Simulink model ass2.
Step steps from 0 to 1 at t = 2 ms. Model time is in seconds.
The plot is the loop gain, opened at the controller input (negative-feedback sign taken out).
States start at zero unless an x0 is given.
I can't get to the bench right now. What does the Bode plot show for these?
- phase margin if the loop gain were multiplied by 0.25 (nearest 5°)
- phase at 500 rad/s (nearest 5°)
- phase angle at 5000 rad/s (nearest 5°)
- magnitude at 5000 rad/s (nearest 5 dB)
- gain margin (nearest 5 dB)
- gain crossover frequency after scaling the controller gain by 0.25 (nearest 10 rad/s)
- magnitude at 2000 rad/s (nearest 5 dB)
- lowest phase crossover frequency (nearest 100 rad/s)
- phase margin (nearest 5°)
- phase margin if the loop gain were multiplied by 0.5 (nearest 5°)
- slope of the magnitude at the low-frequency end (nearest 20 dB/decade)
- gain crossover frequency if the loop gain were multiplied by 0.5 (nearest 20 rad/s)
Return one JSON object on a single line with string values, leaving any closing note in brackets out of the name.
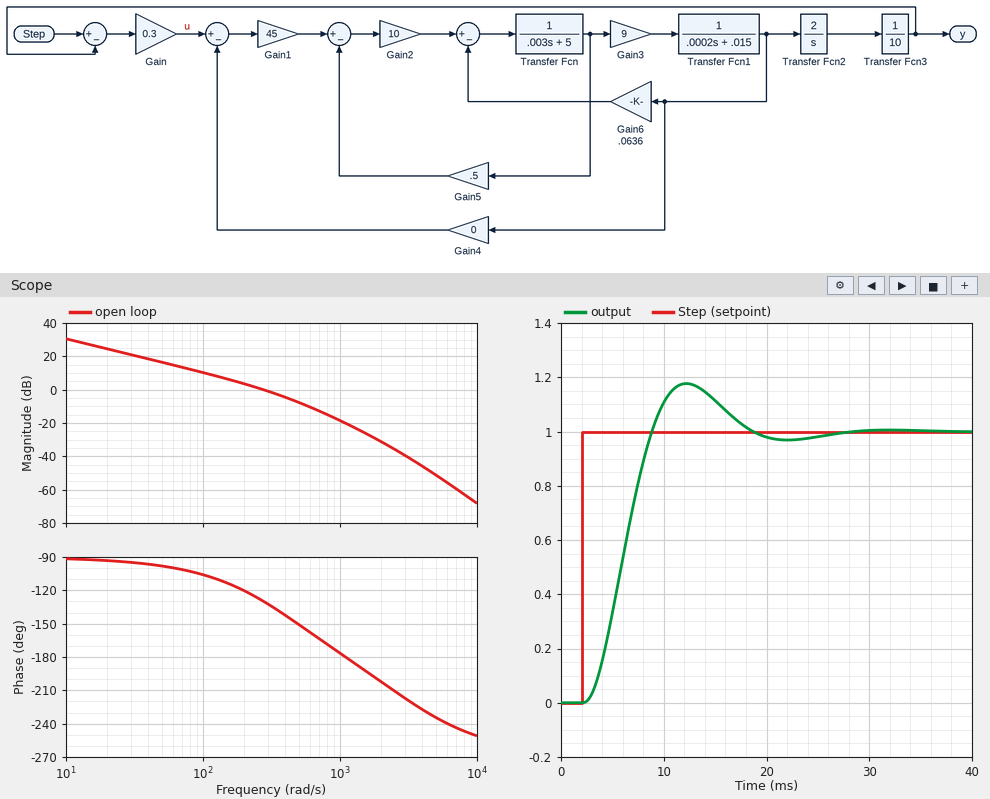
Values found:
{"phase margin if the loop gain were multiplied by 0.25": "75°", "phase at 500 rad/s": "-150°", "phase angle at 5000 rad/s": "-235°", "magnitude at 5000 rad/s": "-50 dB", "gain margin": "20 dB", "gain crossover frequency after scaling the controller gain by 0.25": "80 rad/s", "magnitude at 2000 rad/s": "-30 dB", "lowest phase crossover frequency": "1100 rad/s", "phase margin": "50°", "phase margin if the loop gain were multiplied by 0.5": "65°", "slope of the magnitude at the low-frequency end": "-20 dB/decade", "gain crossover frequency if the loop gain were multiplied by 0.5": "160 rad/s"}
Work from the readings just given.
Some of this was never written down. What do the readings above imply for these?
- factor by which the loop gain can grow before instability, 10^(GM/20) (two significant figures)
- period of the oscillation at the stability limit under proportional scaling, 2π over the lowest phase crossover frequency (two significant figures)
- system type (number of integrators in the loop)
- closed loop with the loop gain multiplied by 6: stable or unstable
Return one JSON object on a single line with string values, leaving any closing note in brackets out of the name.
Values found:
{"factor by which the loop gain can grow before instability, 10^(GM/20)": "10", "period of the oscillation at the stability limit under proportional scaling, 2π over the lowest phase crossover frequency": "0.0057 s", "system type": "1", "closed loop with the loop gain multiplied by 6: stable or unstable": "stable"}
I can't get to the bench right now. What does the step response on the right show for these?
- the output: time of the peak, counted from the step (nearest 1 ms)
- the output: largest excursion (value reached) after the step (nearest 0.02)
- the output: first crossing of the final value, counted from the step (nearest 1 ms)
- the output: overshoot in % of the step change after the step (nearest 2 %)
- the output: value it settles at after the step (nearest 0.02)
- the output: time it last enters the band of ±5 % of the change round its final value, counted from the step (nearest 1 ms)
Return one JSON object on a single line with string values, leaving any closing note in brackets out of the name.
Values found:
{"the output: time of the peak, counted from the step": "10 ms", "the output: largest excursion (value reached) after the step": "1.18", "the output: first crossing of the final value, counted from the step": "7 ms", "the output: overshoot in % of the step change after the step": "18 %", "the output: value it settles at after the step": "1.00", "the output: time it last enters the band of ±5 % of the change round its final value, counted from the step": "15 ms"}
